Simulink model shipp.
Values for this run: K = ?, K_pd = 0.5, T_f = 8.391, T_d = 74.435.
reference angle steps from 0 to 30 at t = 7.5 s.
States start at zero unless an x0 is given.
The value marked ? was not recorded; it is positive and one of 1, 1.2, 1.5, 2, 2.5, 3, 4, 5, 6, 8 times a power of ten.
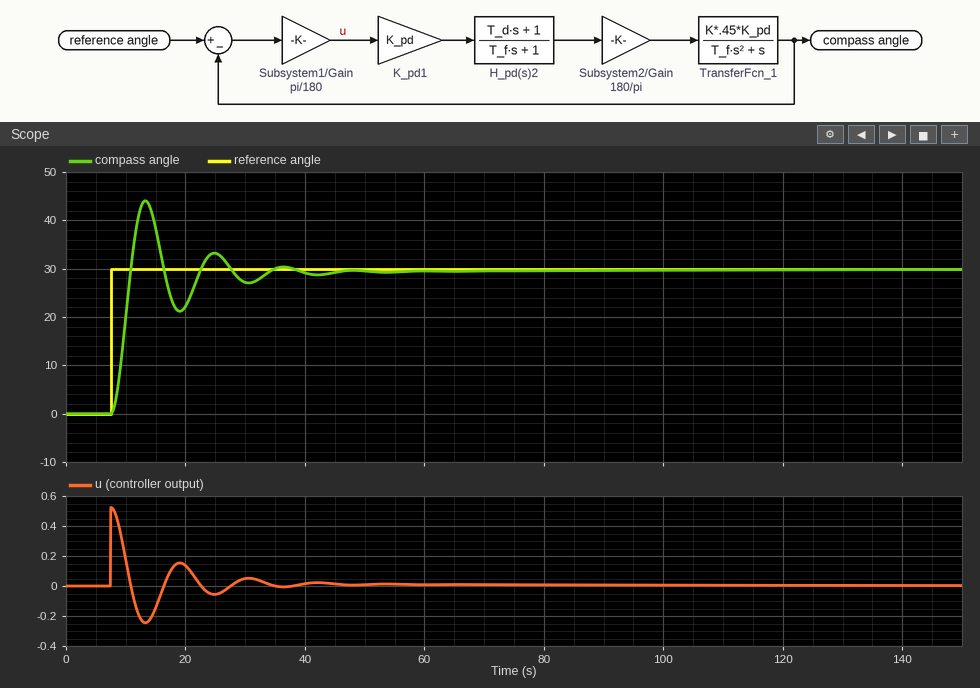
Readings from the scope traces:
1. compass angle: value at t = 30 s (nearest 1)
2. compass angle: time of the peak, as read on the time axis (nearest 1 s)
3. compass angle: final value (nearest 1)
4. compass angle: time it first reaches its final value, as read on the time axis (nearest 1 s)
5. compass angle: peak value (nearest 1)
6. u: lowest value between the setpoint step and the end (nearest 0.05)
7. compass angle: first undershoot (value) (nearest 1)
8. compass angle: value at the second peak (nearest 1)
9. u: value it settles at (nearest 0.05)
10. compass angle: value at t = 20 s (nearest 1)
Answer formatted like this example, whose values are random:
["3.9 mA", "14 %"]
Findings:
["27", "13 s", "30", "11 s", "44", "-0.25", "21", "33", "0.00", "22"]
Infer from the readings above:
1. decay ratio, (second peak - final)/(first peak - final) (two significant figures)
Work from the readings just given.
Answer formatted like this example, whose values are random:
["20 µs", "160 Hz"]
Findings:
["0.21"]
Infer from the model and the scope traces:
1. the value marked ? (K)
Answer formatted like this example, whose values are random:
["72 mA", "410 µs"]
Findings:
["2.5"]
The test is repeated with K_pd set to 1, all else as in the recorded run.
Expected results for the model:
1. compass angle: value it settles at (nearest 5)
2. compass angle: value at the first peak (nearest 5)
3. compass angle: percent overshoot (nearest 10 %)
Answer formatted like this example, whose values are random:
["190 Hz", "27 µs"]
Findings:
["30", "50", "70 %"]
